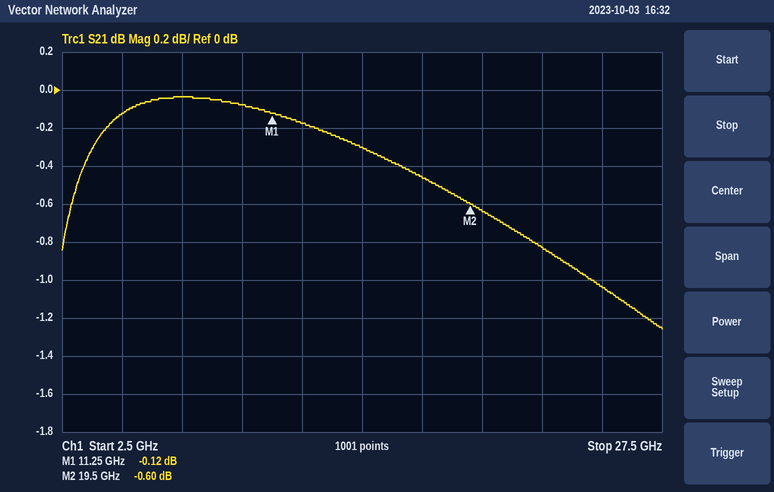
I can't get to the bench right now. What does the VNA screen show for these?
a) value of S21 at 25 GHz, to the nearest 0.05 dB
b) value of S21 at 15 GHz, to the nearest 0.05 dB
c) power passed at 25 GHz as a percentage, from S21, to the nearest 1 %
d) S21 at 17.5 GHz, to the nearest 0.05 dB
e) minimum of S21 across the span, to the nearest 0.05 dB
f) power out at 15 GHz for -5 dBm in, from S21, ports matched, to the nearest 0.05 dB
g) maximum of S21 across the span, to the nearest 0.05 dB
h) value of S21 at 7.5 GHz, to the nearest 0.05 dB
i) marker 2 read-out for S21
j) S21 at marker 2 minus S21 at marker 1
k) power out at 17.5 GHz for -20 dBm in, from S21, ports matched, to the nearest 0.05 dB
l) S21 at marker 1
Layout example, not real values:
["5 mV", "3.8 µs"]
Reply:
["-1.05 dB", "-0.30 dB", "79 %", "-0.45 dB", "-1.25 dB", "-5.30 dBm", "-0.05 dB", "-0.05 dB", "-0.60 dB", "-0.48 dB", "-20.45 dBm", "-0.12 dB"]
